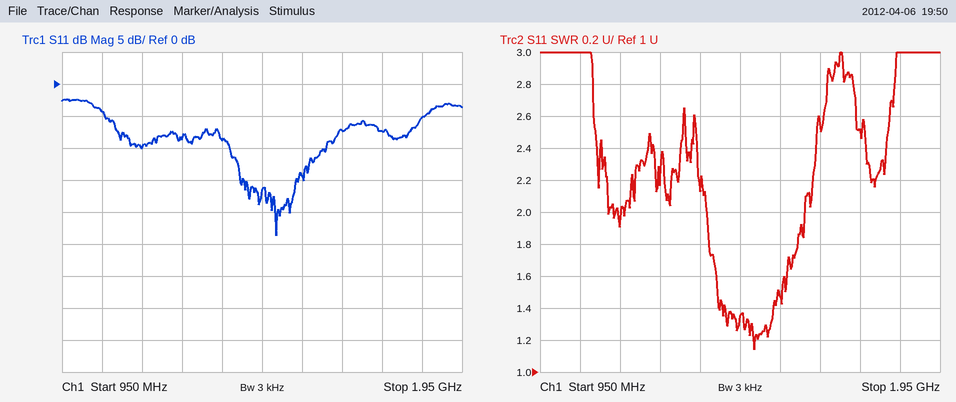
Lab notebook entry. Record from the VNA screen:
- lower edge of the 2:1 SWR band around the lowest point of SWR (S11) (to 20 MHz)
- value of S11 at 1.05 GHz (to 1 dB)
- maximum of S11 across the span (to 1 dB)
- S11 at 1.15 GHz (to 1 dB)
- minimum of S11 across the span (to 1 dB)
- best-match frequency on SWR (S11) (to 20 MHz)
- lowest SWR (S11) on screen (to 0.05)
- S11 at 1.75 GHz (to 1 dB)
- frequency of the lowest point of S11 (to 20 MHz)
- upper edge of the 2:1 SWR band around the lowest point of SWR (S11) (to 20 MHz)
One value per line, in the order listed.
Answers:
1.36 GHz
-4 dB
-2 dB
-10 dB
-24 dB
1.48 GHz
1.15
-7 dB
1.48 GHz
1.62 GHz
